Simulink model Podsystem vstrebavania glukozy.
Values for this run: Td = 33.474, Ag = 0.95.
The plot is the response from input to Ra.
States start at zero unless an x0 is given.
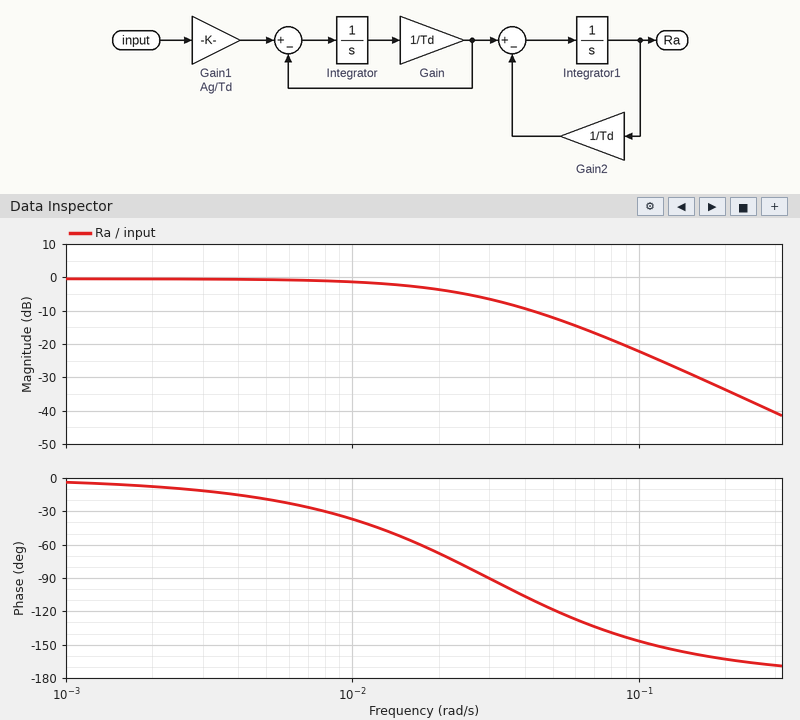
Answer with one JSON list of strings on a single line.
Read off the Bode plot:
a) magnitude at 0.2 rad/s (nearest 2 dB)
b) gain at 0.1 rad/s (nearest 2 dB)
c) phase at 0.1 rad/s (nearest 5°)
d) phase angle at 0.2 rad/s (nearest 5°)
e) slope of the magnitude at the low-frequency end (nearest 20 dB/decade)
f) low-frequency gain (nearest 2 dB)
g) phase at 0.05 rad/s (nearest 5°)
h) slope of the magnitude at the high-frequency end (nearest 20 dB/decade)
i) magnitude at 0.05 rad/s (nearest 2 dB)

["-34 dB", "-22 dB", "-145°", "-165°", "0 dB/decade", "0 dB", "-120°", "-40 dB/decade", "-12 dB"]
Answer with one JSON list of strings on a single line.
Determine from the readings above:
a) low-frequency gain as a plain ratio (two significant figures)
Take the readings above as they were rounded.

["1.0"]
